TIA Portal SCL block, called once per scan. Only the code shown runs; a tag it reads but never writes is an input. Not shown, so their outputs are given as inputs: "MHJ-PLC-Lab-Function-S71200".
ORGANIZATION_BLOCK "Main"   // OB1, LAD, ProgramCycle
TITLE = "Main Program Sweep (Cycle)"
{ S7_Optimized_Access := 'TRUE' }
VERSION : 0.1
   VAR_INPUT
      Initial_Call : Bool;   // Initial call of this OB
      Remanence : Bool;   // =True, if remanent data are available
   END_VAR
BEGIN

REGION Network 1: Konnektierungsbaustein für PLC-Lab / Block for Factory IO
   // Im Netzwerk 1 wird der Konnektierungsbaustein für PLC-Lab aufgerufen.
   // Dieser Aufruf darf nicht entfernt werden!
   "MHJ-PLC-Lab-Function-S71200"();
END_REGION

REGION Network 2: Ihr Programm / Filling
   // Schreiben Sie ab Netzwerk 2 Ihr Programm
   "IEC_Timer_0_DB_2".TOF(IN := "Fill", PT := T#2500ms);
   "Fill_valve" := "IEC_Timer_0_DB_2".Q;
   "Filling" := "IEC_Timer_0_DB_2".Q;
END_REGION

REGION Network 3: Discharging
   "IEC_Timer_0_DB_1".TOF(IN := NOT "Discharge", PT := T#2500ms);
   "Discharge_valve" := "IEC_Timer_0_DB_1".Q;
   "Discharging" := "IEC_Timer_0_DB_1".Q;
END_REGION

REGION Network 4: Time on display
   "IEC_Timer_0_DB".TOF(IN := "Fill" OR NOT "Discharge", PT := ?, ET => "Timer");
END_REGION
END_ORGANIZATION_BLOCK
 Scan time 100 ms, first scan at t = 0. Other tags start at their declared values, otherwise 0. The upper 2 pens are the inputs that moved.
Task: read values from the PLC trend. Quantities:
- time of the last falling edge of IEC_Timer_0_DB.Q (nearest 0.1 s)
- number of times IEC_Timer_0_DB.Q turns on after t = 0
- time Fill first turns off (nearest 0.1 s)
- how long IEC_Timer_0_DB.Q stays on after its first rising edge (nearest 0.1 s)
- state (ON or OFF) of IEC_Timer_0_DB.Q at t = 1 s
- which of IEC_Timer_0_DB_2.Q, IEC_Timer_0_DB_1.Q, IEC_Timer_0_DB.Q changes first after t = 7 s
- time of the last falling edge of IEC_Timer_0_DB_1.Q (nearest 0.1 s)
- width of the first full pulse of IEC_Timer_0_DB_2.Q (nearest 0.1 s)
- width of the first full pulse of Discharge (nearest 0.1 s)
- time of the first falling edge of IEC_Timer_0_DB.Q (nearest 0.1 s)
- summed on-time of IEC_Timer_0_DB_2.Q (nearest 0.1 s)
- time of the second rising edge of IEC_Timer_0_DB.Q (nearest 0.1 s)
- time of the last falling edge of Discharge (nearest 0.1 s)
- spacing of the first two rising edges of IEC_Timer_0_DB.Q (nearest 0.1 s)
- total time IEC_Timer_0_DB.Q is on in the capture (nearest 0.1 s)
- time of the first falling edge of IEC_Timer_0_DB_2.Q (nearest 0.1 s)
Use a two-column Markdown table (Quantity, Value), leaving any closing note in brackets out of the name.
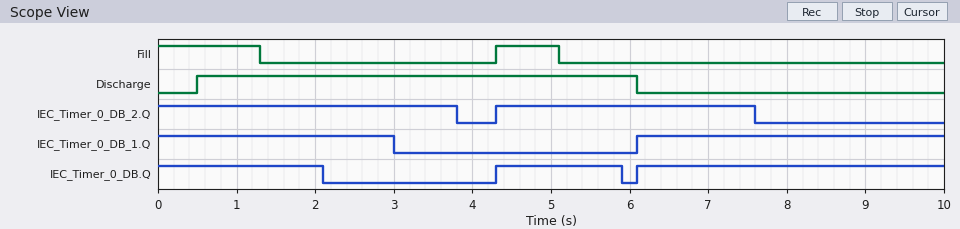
| Quantity | Value |
|---|---|
| time of the last falling edge of IEC_Timer_0_DB.Q | 5.9 s |
| number of times IEC_Timer_0_DB.Q turns on after t = 0 | 2 |
| time Fill first turns off | 1.3 s |
| how long IEC_Timer_0_DB.Q stays on after its first rising edge | 1.6 s |
| state (ON or OFF) of IEC_Timer_0_DB.Q at t = 1 s | ON |
| which of IEC_Timer_0_DB_2.Q, IEC_Timer_0_DB_1.Q, IEC_Timer_0_DB.Q changes first after t = 7 s | IEC_Timer_0_DB_2.Q |
| time of the last falling edge of IEC_Timer_0_DB_1.Q | 3.0 s |
| width of the first full pulse of IEC_Timer_0_DB_2.Q | 3.3 s |
| width of the first full pulse of Discharge | 5.6 s |
| time of the first falling edge of IEC_Timer_0_DB.Q | 2.1 s |
| summed on-time of IEC_Timer_0_DB_2.Q | 7.1 s |
| time of the second rising edge of IEC_Timer_0_DB.Q | 6.1 s |
| time of the last falling edge of Discharge | 6.1 s |
| spacing of the first two rising edges of IEC_Timer_0_DB.Q | 1.8 s |
| total time IEC_Timer_0_DB.Q is on in the capture | 7.6 s |
| time of the first falling edge of IEC_Timer_0_DB_2.Q | 3.8 s |
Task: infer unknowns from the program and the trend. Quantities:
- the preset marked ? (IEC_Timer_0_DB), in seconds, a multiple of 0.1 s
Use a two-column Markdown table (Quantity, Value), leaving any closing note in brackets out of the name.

| Quantity | Value |
|---|---|
| the preset marked ? (IEC_Timer_0_DB), in seconds, a multiple of 0.1 s | 0.8 s |
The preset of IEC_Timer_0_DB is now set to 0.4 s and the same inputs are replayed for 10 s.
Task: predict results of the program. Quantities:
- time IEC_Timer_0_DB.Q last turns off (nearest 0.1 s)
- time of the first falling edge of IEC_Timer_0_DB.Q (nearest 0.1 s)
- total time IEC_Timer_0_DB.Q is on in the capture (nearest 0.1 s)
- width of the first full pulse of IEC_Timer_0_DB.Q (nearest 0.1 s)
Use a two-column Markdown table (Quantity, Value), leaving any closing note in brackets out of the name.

| Quantity | Value |
|---|---|
| time IEC_Timer_0_DB.Q last turns off | 5.5 s |
| time of the first falling edge of IEC_Timer_0_DB.Q | 1.7 s |
| total time IEC_Timer_0_DB.Q is on in the capture | 6.8 s |
| width of the first full pulse of IEC_Timer_0_DB.Q | 1.2 s |
